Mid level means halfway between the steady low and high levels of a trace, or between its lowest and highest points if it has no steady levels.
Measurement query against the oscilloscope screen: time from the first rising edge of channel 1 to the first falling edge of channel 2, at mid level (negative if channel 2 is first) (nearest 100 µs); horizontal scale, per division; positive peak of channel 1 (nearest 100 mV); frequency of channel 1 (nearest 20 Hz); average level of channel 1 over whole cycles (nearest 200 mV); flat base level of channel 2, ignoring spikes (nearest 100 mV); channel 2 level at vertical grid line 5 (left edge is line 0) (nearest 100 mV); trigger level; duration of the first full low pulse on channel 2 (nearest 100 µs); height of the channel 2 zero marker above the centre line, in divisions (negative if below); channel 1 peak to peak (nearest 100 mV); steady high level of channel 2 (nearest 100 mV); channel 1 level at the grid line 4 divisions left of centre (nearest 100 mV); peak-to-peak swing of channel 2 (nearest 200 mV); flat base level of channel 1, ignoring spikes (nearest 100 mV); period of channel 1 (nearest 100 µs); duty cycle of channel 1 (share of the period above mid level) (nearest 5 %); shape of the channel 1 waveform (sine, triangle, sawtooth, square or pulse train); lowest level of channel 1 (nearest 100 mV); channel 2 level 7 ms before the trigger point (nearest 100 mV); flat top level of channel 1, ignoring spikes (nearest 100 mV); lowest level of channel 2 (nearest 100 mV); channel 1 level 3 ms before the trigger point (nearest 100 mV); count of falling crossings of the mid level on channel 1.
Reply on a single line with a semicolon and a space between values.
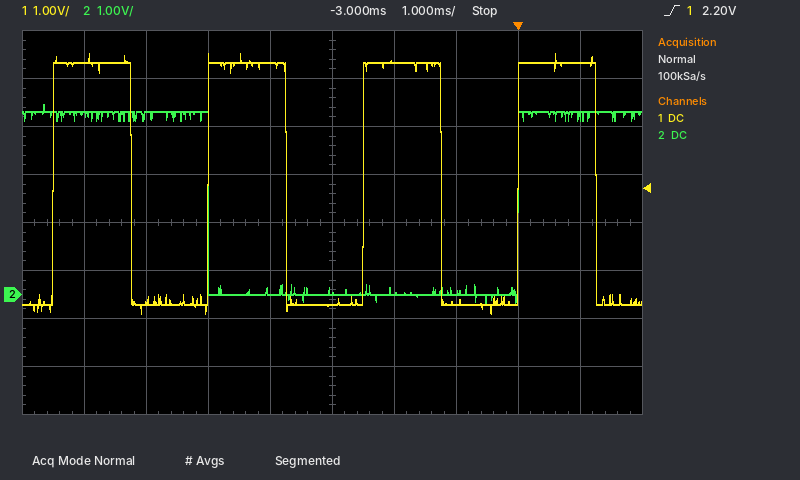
+2.5 ms; 1 ms; 5.0 V; 400 Hz; 2.4 V; 0.0 V; 100 mV; 2.20 V; 5.0 ms; -1.5 div; 5.4 V; 3.8 V; 4.8 V; 4.2 V; -200 mV; 2.5 ms; 50 %; square; -400 mV; 3.8 V; 4.8 V; -200 mV; -200 mV; 4
